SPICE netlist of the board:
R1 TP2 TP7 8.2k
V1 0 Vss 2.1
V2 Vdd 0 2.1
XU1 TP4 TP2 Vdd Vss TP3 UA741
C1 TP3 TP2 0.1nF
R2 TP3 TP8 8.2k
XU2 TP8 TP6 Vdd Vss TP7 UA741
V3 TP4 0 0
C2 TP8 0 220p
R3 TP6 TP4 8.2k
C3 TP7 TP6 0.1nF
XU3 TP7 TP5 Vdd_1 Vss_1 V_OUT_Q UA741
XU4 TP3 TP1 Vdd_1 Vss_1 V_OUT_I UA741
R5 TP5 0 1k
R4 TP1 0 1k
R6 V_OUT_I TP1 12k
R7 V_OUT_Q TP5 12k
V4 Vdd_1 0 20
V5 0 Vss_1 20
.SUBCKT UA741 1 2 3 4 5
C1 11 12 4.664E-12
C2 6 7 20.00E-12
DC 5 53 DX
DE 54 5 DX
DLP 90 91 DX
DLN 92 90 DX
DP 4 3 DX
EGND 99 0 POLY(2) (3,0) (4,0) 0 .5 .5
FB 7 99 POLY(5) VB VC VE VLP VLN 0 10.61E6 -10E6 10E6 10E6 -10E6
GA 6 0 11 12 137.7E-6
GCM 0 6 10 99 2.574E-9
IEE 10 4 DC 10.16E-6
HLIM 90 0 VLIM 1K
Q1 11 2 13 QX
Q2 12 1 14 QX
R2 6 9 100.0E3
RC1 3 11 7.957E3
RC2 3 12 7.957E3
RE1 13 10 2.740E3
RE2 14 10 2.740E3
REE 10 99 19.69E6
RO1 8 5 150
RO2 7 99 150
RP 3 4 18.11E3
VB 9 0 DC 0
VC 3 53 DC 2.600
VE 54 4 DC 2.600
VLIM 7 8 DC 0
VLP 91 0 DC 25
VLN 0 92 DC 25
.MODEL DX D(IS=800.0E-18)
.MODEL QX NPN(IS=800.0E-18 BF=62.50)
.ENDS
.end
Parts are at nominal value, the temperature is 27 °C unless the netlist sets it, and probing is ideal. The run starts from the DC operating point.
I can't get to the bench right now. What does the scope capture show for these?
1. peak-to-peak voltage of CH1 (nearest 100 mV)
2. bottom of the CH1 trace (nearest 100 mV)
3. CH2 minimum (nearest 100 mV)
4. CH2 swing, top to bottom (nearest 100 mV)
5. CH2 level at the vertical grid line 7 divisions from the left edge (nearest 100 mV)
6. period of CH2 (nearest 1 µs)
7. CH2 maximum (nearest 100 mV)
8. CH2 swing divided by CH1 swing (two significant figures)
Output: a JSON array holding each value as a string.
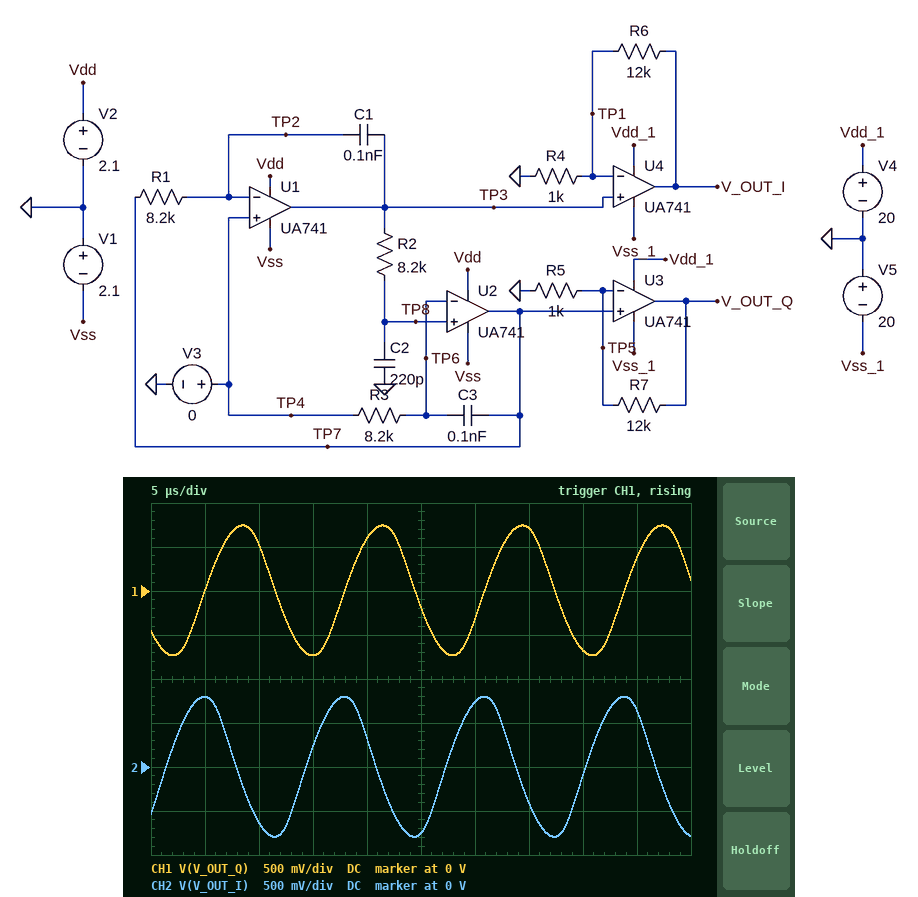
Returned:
["1.5 V", "-700 mV", "-800 mV", "1.6 V", "-400 mV", "13 µs", "800 mV", "1.1"]
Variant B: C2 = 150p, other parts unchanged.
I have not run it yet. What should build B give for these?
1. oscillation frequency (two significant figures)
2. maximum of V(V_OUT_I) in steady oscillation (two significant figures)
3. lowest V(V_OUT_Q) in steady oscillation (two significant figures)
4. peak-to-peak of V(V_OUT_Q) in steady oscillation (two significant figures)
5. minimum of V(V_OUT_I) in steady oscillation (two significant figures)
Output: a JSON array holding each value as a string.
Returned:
["88 kHz", "680 mV", "-640 mV", "1.3 V", "-670 mV"]
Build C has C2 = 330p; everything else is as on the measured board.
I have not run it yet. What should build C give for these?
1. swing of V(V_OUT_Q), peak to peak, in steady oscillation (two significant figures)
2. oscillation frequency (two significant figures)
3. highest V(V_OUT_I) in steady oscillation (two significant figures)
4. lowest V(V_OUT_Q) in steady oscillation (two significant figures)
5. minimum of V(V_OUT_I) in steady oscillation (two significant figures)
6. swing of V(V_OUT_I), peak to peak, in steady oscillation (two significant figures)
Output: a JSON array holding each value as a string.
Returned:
["1.6 V", "67 kHz", "910 mV", "-800 mV", "-900 mV", "1.8 V"]
